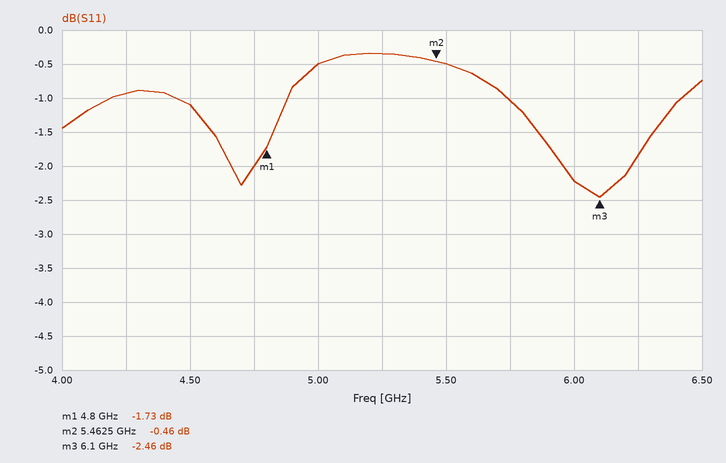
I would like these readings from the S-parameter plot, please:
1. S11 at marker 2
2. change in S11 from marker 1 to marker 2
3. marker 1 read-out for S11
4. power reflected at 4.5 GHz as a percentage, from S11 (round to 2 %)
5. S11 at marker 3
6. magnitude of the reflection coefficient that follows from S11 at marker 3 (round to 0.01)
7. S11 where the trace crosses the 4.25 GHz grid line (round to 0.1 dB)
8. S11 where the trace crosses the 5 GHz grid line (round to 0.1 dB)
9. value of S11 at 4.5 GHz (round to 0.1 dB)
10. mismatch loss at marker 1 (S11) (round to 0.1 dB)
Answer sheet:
-0.46 dB
1.27 dB
-1.73 dB
78 %
-2.46 dB
0.75
-0.9 dB
-0.5 dB
-1.1 dB
4.8 dB
